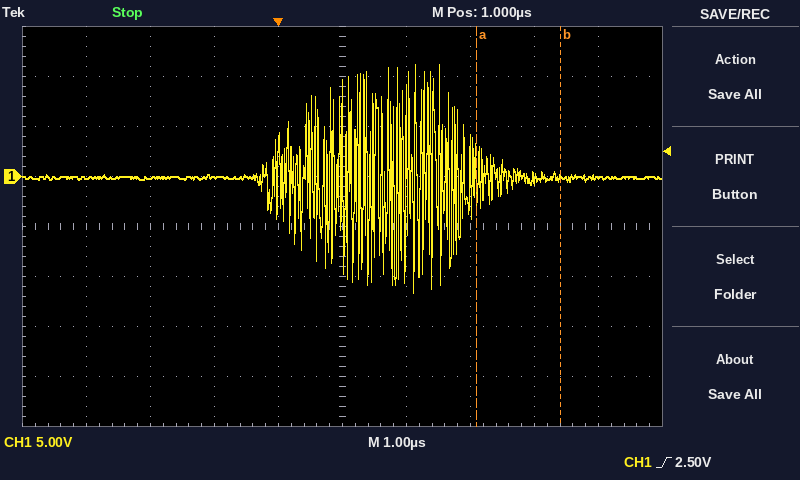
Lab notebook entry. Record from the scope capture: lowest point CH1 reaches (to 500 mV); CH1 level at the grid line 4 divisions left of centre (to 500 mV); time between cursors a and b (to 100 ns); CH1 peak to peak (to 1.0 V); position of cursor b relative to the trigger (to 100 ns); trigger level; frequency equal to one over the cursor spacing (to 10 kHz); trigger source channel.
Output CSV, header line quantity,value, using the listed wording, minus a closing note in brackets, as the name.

quantity,value
lowest point CH1 reaches,-11.5 V
CH1 level at the grid line 4 divisions left of centre,0.0 V
time between cursors a and b,1.3 µs
CH1 peak to peak,23.0 V
position of cursor b relative to the trigger,+4.4 µs
trigger level,2.50 V
frequency equal to one over the cursor spacing,770 kHz
trigger source channel,CH1
